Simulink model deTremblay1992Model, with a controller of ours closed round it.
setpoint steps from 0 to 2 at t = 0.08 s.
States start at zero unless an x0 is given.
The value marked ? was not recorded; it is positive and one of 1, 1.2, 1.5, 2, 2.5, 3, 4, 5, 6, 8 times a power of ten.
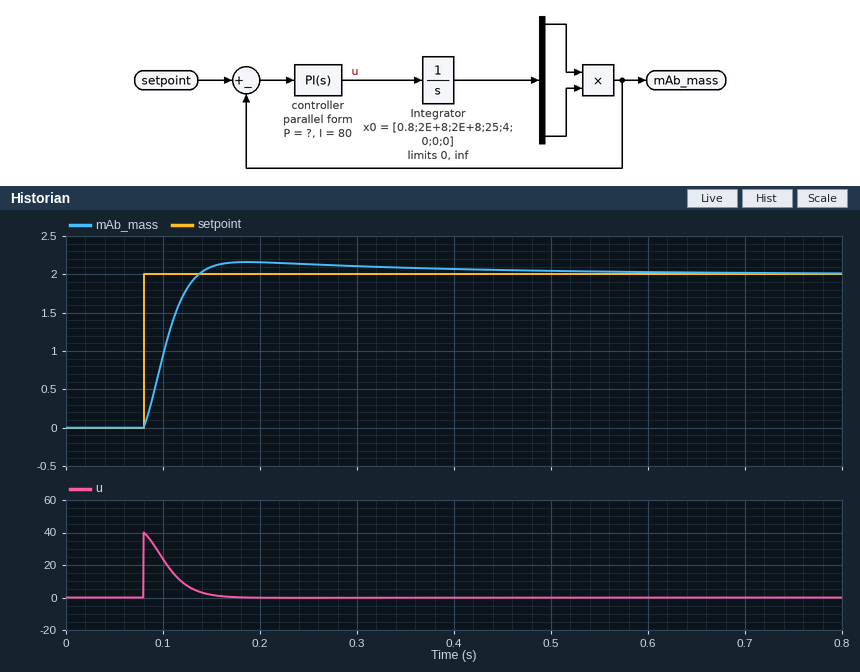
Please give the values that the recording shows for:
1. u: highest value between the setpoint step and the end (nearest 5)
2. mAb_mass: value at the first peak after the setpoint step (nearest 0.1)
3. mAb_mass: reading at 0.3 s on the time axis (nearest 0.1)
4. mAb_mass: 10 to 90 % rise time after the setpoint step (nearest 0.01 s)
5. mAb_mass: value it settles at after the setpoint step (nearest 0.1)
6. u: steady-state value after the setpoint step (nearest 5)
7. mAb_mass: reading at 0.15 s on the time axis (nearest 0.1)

40
2.2
2.1
0.04 s
2.0
0
2.1
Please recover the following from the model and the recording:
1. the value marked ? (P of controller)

20
